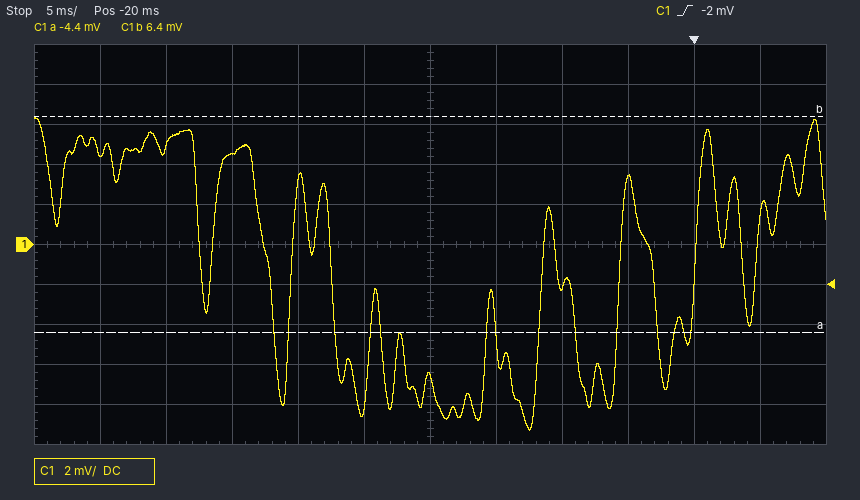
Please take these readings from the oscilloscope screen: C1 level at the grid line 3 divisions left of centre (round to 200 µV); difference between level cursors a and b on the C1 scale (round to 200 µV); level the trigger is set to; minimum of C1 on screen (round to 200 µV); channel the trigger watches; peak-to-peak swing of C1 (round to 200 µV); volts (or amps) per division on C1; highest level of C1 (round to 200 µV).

4.6 mV
10.8 mV
-2 mV
-9.2 mV
C1
15.6 mV
2 mV
6.4 mV
